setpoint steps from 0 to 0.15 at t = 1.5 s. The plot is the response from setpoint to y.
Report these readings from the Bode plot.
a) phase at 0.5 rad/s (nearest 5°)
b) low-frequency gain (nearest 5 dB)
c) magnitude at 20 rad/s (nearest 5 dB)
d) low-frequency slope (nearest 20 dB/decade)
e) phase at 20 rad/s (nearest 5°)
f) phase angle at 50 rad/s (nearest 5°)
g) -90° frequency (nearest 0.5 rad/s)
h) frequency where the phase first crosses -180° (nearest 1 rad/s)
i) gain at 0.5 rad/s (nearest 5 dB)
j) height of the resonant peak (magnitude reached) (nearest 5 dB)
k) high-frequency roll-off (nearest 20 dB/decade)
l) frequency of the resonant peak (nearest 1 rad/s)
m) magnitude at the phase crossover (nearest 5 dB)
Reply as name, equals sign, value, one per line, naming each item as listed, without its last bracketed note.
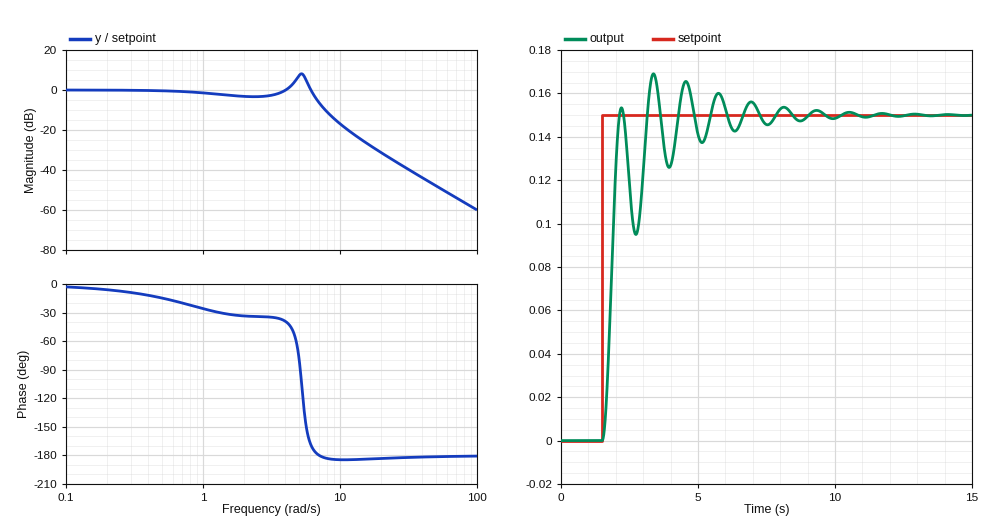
phase at 0.5 rad/s = -15°
low-frequency gain = 0 dB
magnitude at 20 rad/s = -30 dB
low-frequency slope = 0 dB/decade
phase at 20 rad/s = -185°
phase angle at 50 rad/s = -180°
-90° frequency = 5.0 rad/s
frequency where the phase first crosses -180° = 7 rad/s
gain at 0.5 rad/s = 0 dB
height of the resonant peak (magnitude reached) = 10 dB
high-frequency roll-off = -40 dB/decade
frequency of the resonant peak = 5 rad/s
magnitude at the phase crossover = -5 dB
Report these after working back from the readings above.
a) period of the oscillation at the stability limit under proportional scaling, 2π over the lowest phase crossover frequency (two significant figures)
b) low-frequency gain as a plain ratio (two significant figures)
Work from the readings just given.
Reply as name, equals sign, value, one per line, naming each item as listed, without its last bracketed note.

period of the oscillation at the stability limit under proportional scaling, 2π over the lowest phase crossover frequency = 0.90 s
low-frequency gain as a plain ratio = 1.0
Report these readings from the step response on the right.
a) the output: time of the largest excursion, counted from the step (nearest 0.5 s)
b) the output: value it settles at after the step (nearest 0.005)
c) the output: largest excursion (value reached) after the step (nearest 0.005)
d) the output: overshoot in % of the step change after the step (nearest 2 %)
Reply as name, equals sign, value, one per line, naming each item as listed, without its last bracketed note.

the output: time of the largest excursion, counted from the step = 2.0 s
the output: value it settles at after the step = 0.150
the output: largest excursion (value reached) after the step = 0.170
the output: overshoot in % of the step change after the step = 12 %
